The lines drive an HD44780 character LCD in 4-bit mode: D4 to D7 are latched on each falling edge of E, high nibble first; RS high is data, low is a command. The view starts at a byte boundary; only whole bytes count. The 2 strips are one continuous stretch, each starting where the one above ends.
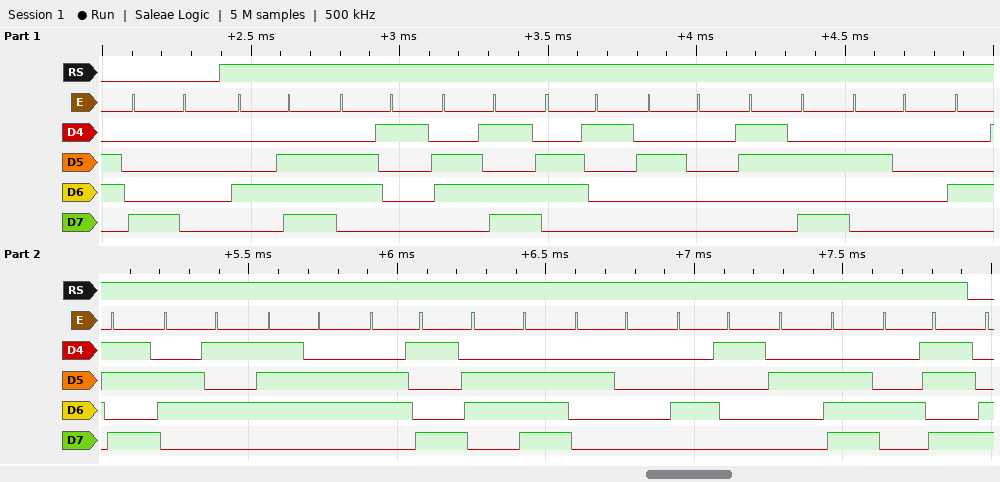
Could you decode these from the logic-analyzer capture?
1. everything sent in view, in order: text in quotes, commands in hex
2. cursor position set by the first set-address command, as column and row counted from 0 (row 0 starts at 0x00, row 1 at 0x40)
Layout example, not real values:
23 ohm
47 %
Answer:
0x80 "Nama : Kevin A.K"
column 0, row 0
